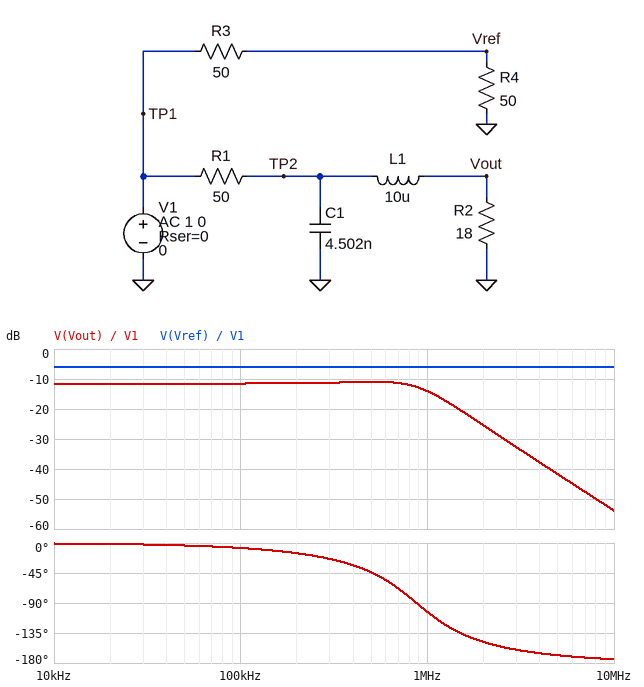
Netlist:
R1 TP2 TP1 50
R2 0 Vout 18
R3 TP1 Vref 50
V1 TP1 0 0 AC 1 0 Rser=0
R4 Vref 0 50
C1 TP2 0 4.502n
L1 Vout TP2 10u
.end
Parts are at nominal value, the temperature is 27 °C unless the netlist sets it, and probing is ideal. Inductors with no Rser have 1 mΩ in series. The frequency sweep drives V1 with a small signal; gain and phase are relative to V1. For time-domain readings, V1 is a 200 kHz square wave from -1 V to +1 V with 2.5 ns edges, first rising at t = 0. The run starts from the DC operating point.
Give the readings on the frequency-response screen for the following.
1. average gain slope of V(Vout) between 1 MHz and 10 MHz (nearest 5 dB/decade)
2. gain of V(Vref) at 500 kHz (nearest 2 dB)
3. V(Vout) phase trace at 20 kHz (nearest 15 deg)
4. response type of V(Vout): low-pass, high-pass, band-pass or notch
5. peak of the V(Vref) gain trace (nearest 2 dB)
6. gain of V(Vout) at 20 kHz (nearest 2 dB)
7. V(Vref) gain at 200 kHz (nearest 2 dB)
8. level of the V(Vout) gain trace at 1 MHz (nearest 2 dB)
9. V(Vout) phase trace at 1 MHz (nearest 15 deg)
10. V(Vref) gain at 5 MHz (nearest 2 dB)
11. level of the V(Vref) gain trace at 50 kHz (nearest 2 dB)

-40 dB/decade
-6 dB
0 deg
low-pass
-6 dB
-12 dB
-6 dB
-14 dB
-105 deg
-6 dB
-6 dB
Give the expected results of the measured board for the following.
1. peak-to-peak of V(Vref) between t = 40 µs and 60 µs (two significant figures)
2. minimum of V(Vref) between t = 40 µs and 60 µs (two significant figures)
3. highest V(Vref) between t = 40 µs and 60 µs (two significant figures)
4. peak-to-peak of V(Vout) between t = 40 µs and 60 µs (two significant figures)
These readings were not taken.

1.0 V
-500 mV
500 mV
650 mV
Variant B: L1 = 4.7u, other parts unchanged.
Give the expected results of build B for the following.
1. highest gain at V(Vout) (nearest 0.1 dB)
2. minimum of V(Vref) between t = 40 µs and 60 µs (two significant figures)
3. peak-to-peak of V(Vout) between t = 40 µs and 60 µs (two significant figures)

-10.5 dB
-500 mV
690 mV
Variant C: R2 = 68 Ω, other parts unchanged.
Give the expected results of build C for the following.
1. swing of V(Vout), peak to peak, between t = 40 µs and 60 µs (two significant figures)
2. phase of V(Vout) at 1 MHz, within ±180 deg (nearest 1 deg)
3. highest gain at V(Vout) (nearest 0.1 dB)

1.2 V
-80 deg
-4.8 dB
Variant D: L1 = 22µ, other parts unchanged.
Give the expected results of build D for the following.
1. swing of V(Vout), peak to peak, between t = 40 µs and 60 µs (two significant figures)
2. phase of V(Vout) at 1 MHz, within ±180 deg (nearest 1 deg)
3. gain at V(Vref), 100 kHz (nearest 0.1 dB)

570 mV
-128 deg
-6.0 dB
